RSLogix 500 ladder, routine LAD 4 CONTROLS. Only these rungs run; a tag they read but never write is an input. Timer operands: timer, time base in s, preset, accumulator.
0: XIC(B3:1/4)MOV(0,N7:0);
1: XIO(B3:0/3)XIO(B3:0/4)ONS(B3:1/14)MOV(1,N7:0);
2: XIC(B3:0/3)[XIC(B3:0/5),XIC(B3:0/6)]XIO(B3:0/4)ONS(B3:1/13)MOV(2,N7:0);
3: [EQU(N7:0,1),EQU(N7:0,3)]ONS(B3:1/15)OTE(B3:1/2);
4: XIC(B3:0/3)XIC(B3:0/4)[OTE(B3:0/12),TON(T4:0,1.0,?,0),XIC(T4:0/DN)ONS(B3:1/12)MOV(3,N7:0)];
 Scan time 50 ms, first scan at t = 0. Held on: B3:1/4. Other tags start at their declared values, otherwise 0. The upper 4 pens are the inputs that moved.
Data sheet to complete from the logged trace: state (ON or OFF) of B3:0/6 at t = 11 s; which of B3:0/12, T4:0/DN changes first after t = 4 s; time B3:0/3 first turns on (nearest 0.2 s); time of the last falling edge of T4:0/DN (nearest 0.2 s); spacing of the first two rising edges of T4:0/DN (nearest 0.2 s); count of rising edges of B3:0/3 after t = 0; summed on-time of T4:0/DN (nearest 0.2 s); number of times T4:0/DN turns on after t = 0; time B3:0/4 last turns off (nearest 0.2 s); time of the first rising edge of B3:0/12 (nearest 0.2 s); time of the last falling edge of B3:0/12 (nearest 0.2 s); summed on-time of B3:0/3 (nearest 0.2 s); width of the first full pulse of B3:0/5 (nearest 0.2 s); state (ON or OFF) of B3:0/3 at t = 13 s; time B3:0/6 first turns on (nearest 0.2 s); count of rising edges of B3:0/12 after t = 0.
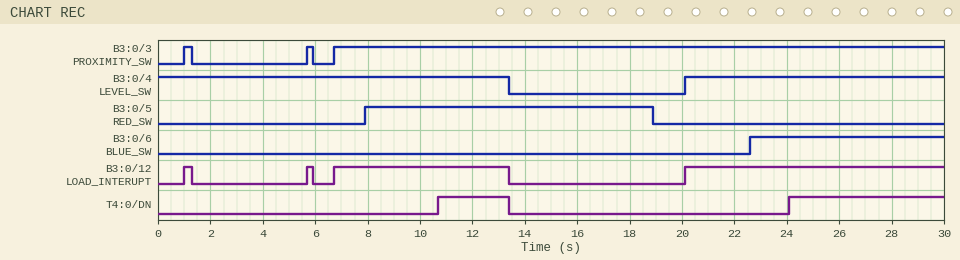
OFF
B3:0/12
1.0 s
13.4 s
13.4 s
3
8.6 s
2
13.4 s
1.0 s
13.4 s
23.8 s
11.0 s
ON
22.6 s
4
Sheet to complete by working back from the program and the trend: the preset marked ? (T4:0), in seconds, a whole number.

4 s
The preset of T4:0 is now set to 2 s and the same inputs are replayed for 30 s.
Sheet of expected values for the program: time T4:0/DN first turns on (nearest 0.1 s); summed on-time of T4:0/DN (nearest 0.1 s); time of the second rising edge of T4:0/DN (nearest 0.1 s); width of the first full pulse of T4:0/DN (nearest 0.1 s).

8.7 s
12.6 s
22.1 s
4.7 s
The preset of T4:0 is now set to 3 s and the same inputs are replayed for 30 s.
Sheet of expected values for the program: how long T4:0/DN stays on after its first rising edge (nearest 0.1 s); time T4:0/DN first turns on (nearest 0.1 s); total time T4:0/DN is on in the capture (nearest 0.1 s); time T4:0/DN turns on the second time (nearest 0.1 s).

3.7 s
9.7 s
10.6 s
23.1 s
